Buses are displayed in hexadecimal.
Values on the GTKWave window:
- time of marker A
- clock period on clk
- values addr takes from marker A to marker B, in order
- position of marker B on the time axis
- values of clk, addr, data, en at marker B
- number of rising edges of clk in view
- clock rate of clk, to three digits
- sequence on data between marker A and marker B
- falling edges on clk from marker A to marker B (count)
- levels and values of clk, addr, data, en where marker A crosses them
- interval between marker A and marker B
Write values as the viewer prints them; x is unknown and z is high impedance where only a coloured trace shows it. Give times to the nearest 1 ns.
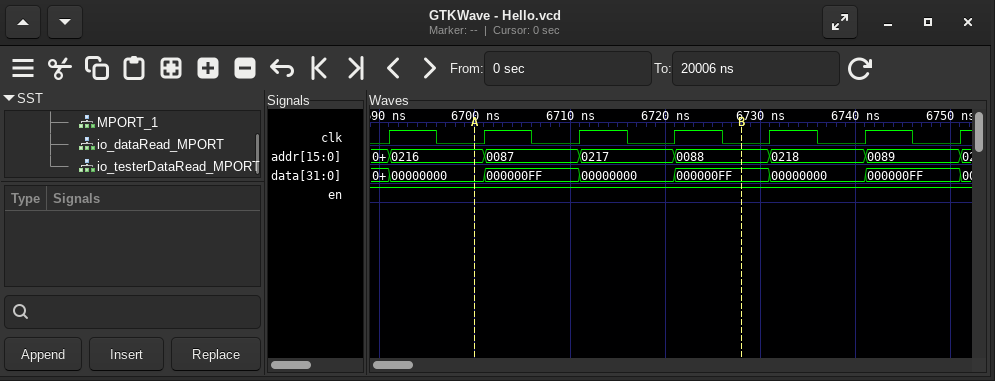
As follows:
6700 ns
10 ns
0216, 0087, 0217, 0088
6728 ns
clk=0, addr=0088, data=000000FF, en=1
7
100 MHz
00000000, 000000FF, 00000000, 000000FF
3
clk=0, addr=0216, data=00000000, en=1
28 ns
